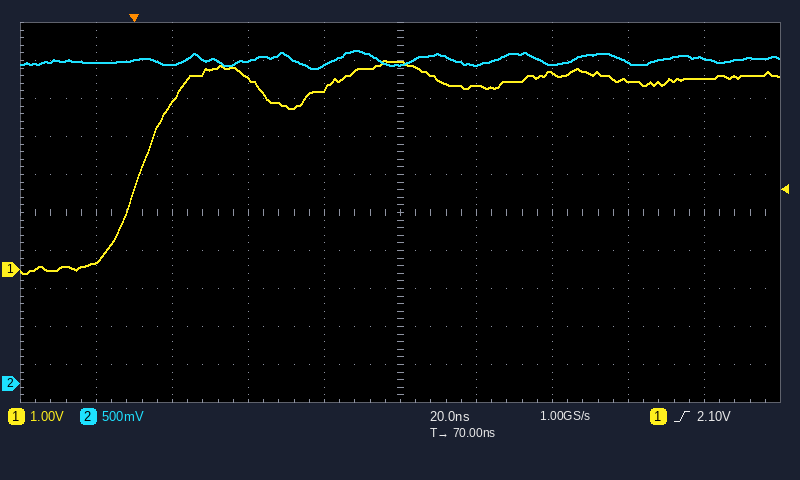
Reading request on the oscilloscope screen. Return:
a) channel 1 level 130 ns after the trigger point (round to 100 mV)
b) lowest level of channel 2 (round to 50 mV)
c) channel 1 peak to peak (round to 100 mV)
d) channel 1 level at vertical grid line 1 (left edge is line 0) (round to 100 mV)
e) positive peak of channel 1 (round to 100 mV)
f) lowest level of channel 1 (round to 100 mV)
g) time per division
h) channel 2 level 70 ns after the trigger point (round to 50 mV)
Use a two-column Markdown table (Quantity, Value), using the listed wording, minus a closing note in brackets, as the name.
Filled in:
| Quantity | Value |
|---|---|
| channel 1 level 130 ns after the trigger point | 5.0 V |
| lowest level of channel 2 | 4.15 V |
| channel 1 peak to peak | 5.6 V |
| channel 1 level at vertical grid line 1 (left edge is line 0) | 200 mV |
| positive peak of channel 1 | 5.5 V |
| lowest level of channel 1 | -100 mV |
| time per division | 20 ns |
| channel 2 level 70 ns after the trigger point | 4.20 V |
